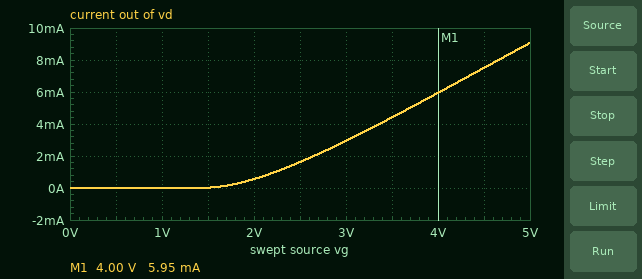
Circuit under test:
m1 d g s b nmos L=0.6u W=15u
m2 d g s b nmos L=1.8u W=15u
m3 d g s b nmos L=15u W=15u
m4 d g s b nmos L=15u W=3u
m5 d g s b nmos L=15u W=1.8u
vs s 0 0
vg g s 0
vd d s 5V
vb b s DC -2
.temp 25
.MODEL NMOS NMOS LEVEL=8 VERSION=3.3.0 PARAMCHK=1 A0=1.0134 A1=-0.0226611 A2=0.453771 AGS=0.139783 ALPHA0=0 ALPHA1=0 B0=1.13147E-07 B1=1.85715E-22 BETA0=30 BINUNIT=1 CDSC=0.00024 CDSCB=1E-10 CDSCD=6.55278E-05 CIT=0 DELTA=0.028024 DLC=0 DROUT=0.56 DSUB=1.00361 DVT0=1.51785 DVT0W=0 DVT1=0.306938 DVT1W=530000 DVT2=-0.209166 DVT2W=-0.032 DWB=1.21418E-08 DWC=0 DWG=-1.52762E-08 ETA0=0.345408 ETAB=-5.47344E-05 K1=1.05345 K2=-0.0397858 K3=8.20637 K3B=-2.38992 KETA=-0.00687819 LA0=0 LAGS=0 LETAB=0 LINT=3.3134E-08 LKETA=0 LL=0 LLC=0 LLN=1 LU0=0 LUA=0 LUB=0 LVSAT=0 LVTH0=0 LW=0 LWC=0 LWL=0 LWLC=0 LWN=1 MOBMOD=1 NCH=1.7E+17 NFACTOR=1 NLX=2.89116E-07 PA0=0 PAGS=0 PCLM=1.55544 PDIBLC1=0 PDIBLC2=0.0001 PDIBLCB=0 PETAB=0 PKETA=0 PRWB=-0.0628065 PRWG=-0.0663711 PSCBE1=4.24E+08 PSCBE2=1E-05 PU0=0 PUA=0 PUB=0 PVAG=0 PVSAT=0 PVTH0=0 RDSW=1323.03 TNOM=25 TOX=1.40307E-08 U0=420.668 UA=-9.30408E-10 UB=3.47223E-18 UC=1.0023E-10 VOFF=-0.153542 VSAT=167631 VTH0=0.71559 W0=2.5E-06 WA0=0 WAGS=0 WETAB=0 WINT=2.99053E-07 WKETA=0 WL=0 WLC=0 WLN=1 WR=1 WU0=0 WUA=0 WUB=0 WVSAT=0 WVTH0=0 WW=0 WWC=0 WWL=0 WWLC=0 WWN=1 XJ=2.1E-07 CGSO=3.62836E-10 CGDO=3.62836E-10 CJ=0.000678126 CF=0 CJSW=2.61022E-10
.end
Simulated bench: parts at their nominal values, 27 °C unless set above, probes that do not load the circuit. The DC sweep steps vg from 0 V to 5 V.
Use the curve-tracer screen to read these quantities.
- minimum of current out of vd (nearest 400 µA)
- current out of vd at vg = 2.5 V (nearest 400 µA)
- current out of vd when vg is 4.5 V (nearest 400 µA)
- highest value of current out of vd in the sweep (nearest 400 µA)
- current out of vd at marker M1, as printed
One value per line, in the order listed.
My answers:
0 A
1.6 mA
7.6 mA
9.2 mA
5.95 mA
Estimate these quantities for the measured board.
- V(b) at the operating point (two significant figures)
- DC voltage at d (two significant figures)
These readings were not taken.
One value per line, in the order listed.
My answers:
-2.0 V
5.0 V
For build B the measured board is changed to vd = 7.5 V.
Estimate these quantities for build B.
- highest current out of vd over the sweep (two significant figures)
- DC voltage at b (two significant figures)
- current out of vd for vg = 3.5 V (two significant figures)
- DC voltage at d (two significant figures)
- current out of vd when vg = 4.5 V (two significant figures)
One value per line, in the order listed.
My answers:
10 mA
-2.0 V
5.4 mA
7.5 V
8.7 mA
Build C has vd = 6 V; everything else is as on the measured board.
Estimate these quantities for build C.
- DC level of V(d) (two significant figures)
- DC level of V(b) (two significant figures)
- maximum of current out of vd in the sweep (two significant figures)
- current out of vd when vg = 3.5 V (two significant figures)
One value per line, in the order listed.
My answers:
6.0 V
-2.0 V
9.2 mA
4.5 mA
